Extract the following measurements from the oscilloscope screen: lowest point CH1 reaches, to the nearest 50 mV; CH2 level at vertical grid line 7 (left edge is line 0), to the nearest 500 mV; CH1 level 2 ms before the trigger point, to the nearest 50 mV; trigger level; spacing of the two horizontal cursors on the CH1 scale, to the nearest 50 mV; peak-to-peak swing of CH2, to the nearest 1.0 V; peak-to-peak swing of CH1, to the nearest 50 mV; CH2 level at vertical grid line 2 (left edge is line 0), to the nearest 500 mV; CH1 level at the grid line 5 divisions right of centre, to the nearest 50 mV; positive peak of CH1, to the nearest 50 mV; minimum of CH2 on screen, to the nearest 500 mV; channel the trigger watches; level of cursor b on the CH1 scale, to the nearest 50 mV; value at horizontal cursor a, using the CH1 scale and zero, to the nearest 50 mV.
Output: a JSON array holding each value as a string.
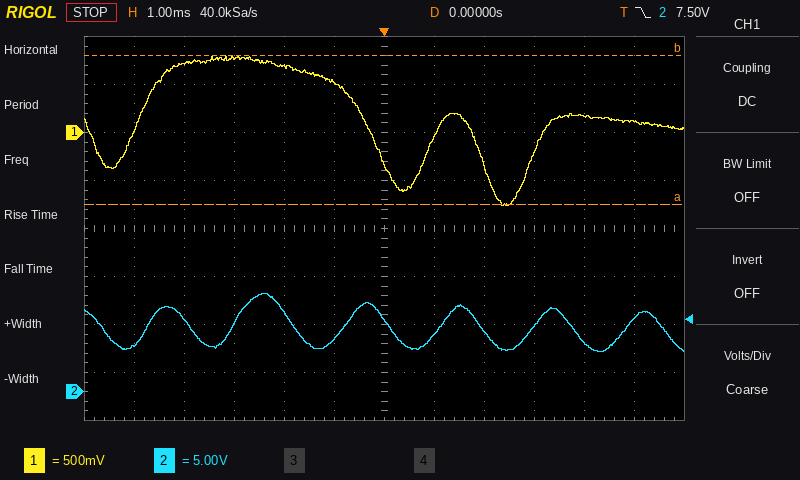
["-750 mV", "6.0 V", "700 mV", "7.50 V", "1.55 V", "6.0 V", "1.55 V", "7.5 V", "100 mV", "800 mV", "4.0 V", "CH2", "800 mV", "-750 mV"]
